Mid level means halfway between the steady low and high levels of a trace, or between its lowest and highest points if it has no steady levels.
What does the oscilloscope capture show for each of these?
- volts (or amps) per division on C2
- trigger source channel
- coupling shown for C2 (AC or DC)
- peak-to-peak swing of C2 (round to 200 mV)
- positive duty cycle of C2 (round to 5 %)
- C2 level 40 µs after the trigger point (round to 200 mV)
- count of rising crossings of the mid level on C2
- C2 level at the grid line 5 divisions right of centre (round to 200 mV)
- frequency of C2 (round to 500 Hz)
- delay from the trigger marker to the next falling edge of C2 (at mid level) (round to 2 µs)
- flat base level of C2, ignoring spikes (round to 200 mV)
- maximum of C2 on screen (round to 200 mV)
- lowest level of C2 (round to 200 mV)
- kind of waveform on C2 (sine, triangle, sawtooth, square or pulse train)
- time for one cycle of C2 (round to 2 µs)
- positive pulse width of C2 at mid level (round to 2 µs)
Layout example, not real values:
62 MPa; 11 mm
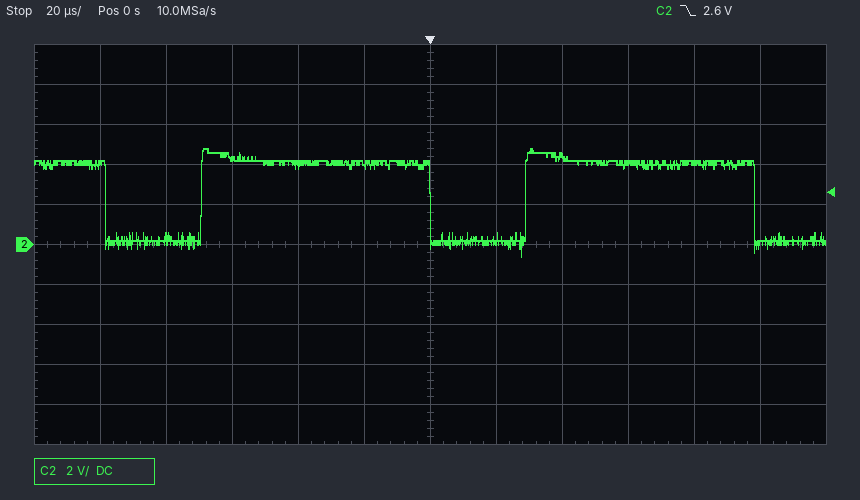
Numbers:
2 V; C2; DC; 5.4 V; 70 %; 4.4 V; 2; 0.0 V; 10.0 kHz; 98 µs; 200 mV; 4.8 V; -600 mV; pulse train; 98 µs; 70 µs
